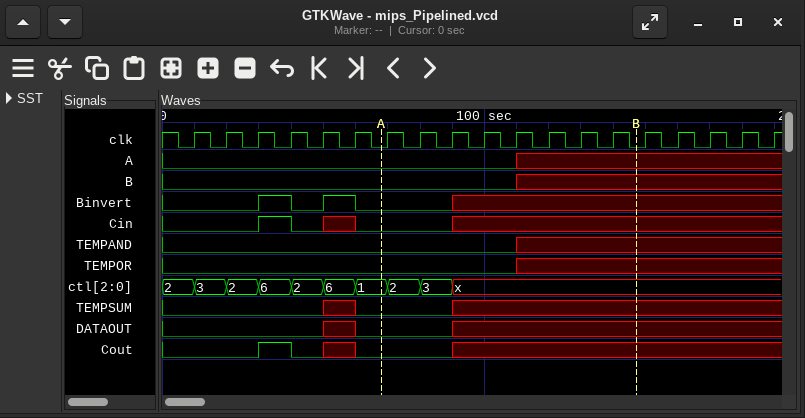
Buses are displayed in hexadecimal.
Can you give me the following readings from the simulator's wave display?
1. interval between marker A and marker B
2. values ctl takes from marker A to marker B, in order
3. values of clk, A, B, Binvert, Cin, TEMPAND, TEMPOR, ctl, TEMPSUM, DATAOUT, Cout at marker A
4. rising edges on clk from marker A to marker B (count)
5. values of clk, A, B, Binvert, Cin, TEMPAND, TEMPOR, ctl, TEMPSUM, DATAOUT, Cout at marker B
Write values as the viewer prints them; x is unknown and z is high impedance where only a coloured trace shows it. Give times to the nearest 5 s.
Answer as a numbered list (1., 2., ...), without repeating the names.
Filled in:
1. 80 s
2. 1, 2, 3, x
3. clk=0, A=0, B=0, Binvert=0, Cin=0, TEMPAND=0, TEMPOR=0, ctl=1, TEMPSUM=0, DATAOUT=0, Cout=0
4. 8
5. clk=0, A=x, B=x, Binvert=x, Cin=x, TEMPAND=x, TEMPOR=x, ctl=x, TEMPSUM=x, DATAOUT=x, Cout=x
